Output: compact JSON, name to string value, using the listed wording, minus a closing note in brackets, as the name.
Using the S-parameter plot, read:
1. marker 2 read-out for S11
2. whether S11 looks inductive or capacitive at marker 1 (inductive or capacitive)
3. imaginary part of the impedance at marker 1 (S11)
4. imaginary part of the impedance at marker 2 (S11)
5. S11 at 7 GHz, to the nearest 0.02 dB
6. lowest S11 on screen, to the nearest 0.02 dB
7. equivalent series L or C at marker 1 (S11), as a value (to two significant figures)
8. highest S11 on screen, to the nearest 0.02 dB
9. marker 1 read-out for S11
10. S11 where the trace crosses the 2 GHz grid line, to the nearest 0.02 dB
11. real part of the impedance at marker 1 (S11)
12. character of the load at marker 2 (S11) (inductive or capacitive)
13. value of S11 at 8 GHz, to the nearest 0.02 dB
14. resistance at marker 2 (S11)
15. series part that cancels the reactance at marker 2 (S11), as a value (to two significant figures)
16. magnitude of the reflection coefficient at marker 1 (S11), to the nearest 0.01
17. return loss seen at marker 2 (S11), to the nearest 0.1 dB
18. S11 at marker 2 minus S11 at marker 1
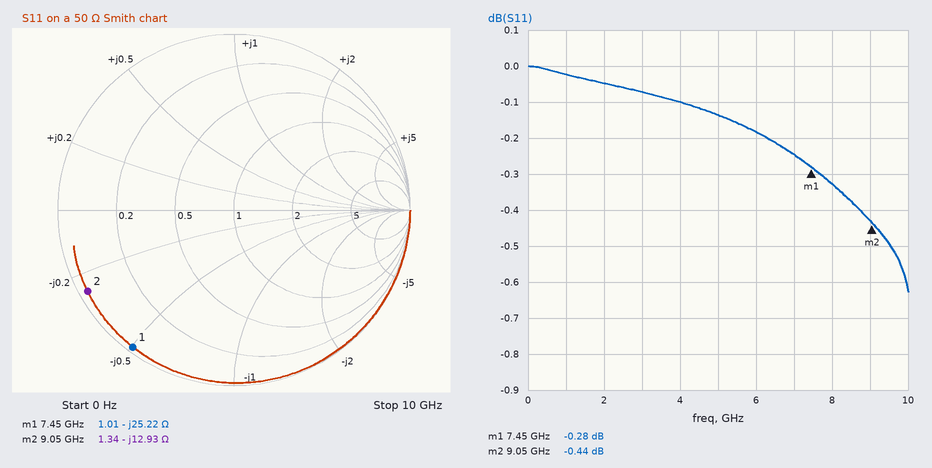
{"marker 2 read-out for S11": "-0.44 dB", "whether S11 looks inductive or capacitive at marker 1": "capacitive", "imaginary part of the impedance at marker 1": "-25.22 Ω", "imaginary part of the impedance at marker 2": "-12.93 Ω", "S11 at 7 GHz, to the nearest 0.02 dB": "-0.24 dB", "lowest S11 on screen, to the nearest 0.02 dB": "-0.62 dB", "equivalent series L or C at marker 1 (S11), as a value": "850 fF", "highest S11 on screen, to the nearest 0.02 dB": "0.00 dB", "marker 1 read-out for S11": "-0.28 dB", "S11 where the trace crosses the 2 GHz grid line, to the nearest 0.02 dB": "-0.04 dB", "real part of the impedance at marker 1": "1.01 Ω", "character of the load at marker 2 (S11)": "capacitive", "value of S11 at 8 GHz, to the nearest 0.02 dB": "-0.32 dB", "resistance at marker 2": "1.34 Ω", "series part that cancels the reactance at marker 2 (S11), as a value": "230 pH", "magnitude of the reflection coefficient at marker 1 (S11), to the nearest 0.01": "0.97", "return loss seen at marker 2 (S11), to the nearest 0.1 dB": "0.4 dB", "S11 at marker 2 minus S11 at marker 1": "-0.16 dB"}
